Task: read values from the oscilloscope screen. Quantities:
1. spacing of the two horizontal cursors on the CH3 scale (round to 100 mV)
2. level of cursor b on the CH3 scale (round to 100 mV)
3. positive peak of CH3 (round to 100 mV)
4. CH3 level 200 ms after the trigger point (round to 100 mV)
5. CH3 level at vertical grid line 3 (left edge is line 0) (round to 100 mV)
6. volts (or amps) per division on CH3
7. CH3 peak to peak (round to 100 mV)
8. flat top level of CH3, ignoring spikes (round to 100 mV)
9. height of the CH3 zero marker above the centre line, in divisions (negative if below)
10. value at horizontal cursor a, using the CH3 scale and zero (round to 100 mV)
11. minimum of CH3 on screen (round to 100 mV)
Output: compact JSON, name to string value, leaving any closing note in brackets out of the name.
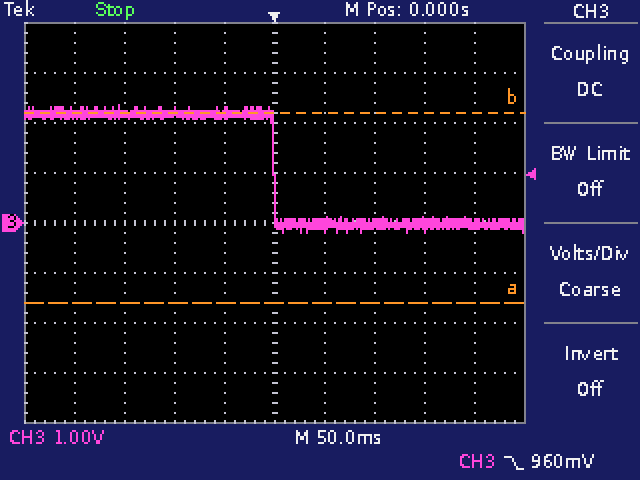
{"spacing of the two horizontal cursors on the CH3 scale": "3.8 V", "level of cursor b on the CH3 scale": "2.2 V", "positive peak of CH3": "2.4 V", "CH3 level 200 ms after the trigger point": "0.0 V", "CH3 level at vertical grid line 3 (left edge is line 0)": "2.2 V", "volts (or amps) per division on CH3": "1 V", "CH3 peak to peak": "2.6 V", "flat top level of CH3, ignoring spikes": "2.2 V", "height of the CH3 zero marker above the centre line, in divisions": "0.0 div", "value at horizontal cursor a, using the CH3 scale and zero": "-1.6 V", "minimum of CH3 on screen": "-200 mV"}
